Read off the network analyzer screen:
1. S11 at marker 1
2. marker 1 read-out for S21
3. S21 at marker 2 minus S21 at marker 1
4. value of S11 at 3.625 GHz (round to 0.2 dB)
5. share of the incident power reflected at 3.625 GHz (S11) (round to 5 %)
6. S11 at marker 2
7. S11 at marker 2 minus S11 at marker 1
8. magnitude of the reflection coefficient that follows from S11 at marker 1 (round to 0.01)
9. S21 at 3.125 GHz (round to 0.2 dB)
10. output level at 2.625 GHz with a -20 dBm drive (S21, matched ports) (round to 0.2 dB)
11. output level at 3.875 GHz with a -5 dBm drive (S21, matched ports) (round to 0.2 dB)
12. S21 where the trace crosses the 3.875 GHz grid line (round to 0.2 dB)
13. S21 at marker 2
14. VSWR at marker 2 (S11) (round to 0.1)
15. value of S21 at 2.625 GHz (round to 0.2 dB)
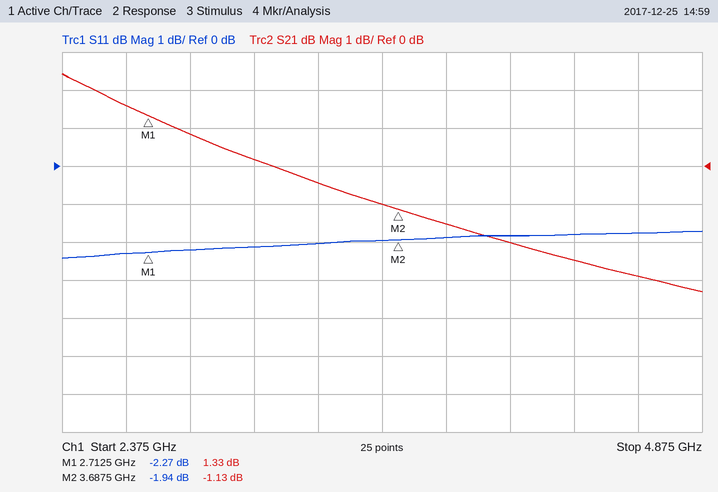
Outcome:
-2.27 dB
1.33 dB
-2.46 dB
-2.0 dB
65 %
-1.94 dB
0.33 dB
0.77
0.2 dB
-18.4 dBm
-6.6 dBm
-1.6 dB
-1.13 dB
9.0
1.6 dB
